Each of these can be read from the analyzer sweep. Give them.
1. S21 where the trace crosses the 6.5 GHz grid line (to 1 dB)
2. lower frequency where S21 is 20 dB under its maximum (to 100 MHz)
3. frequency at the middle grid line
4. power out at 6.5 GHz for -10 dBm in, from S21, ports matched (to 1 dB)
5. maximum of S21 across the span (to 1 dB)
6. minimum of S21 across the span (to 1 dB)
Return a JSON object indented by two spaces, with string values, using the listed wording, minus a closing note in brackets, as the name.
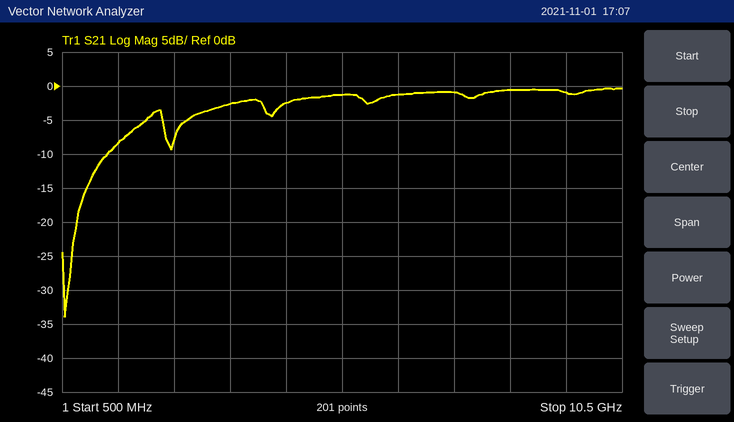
{
  "S21 where the trace crosses the 6.5 GHz grid line": "-1 dB",
  "lower frequency where S21 is 20 dB under its maximum": "800 MHz",
  "frequency at the middle grid line": "5.5 GHz",
  "power out at 6.5 GHz for -10 dBm in, from S21, ports matched": "-11 dBm",
  "maximum of S21 across the span": "0 dB",
  "minimum of S21 across the span": "-34 dB"
}
